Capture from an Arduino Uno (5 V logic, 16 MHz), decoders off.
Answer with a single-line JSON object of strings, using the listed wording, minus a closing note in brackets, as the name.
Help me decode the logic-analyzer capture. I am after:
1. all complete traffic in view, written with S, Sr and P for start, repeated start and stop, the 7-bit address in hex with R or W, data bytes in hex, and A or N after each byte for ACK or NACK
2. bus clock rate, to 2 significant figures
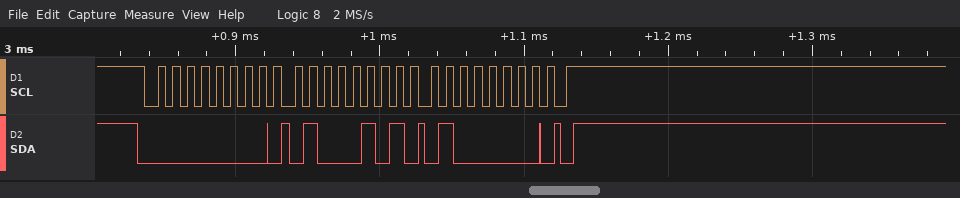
{"all complete traffic in view, written with S, Sr and P for start, repeated start and stop, the 7-bit address in hex with R or W, data bytes in hex, and A or N after each byte for ACK or NACK": "S 00W A 45 A 40 A P", "bus clock rate, to 2 significant figures": "100 kHz"}
